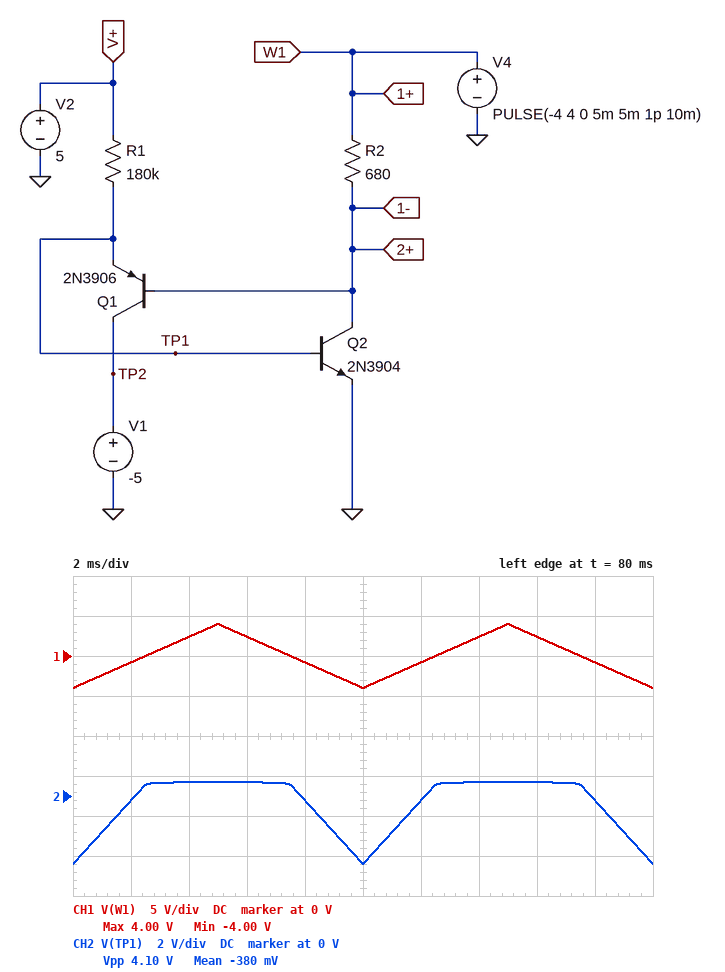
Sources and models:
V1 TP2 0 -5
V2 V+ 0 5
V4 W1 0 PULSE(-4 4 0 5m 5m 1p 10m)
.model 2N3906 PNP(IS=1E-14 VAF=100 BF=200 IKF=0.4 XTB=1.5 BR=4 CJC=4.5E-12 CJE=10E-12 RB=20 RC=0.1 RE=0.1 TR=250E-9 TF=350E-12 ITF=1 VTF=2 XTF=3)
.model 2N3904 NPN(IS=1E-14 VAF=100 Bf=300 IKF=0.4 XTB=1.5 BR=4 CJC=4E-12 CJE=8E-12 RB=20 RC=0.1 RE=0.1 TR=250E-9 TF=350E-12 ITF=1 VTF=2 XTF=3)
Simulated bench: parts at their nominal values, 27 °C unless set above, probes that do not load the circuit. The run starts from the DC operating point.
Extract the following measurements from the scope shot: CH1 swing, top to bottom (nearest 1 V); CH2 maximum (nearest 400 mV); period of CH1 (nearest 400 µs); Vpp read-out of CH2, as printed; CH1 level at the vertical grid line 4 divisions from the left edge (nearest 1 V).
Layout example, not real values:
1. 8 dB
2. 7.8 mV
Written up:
1. 8 V
2. 800 mV
3. 10.0 ms
4. 4.10 V
5. -1 V
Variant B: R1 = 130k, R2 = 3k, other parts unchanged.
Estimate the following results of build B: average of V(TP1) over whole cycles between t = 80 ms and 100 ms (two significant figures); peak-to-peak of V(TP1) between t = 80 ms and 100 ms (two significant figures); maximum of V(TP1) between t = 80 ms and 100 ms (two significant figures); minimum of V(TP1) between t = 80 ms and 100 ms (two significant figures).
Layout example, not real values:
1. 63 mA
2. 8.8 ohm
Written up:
1. -330 mV
2. 3.9 V
3. 660 mV
4. -3.2 V
